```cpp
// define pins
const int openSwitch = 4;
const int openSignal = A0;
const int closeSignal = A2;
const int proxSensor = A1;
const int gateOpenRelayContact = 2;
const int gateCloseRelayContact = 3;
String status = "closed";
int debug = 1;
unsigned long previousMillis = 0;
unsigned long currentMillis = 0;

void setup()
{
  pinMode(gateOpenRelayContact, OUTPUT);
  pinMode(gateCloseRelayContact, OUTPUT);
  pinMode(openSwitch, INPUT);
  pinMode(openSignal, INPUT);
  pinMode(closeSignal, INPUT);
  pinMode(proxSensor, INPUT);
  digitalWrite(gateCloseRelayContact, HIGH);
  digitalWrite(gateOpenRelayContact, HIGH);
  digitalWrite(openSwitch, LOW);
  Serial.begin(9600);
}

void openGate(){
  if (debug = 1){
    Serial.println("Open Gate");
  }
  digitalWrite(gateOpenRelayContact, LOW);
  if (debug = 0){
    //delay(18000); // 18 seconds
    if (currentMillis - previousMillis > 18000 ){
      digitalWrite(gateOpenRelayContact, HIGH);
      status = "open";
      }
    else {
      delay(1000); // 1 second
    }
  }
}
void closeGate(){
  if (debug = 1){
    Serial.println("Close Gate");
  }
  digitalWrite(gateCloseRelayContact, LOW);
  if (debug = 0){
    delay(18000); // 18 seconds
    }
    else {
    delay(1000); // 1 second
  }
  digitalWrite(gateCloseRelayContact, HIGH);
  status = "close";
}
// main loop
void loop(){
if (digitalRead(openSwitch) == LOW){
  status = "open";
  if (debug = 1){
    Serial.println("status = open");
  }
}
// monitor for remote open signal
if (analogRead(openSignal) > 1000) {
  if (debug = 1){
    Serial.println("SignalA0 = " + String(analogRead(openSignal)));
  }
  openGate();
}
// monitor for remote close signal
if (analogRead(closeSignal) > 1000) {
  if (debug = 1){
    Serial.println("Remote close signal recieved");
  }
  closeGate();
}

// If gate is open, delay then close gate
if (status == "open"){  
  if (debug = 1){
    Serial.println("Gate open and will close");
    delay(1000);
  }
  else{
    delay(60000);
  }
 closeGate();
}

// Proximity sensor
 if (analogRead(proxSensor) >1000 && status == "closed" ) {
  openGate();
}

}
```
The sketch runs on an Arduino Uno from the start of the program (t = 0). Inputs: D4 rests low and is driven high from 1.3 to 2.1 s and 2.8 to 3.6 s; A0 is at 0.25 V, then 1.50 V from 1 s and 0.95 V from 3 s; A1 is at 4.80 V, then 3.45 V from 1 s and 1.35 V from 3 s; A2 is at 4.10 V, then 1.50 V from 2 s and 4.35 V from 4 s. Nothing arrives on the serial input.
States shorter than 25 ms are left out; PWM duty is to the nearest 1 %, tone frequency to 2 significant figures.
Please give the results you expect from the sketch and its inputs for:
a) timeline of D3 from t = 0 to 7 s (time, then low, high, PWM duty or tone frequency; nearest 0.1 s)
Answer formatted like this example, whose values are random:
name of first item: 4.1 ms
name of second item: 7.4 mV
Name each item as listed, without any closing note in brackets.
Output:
timeline of D3 from t = 0 to 7 s: 0 s high; 1 s low; 2 s high; 3.1 s low; 4.1 s high; 5.1 s low; 6.1 s high
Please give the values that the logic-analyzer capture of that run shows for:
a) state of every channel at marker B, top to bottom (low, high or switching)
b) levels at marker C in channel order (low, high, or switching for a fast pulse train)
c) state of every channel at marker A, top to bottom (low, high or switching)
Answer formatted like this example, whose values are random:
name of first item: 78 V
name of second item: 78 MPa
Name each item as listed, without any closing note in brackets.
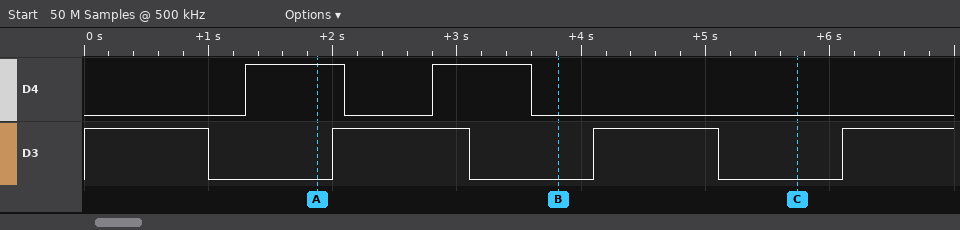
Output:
state of every channel at marker B, top to bottom: D4 low, D3 low
levels at marker C in channel order: D4 low, D3 low
state of every channel at marker A, top to bottom: D4 high, D3 low
